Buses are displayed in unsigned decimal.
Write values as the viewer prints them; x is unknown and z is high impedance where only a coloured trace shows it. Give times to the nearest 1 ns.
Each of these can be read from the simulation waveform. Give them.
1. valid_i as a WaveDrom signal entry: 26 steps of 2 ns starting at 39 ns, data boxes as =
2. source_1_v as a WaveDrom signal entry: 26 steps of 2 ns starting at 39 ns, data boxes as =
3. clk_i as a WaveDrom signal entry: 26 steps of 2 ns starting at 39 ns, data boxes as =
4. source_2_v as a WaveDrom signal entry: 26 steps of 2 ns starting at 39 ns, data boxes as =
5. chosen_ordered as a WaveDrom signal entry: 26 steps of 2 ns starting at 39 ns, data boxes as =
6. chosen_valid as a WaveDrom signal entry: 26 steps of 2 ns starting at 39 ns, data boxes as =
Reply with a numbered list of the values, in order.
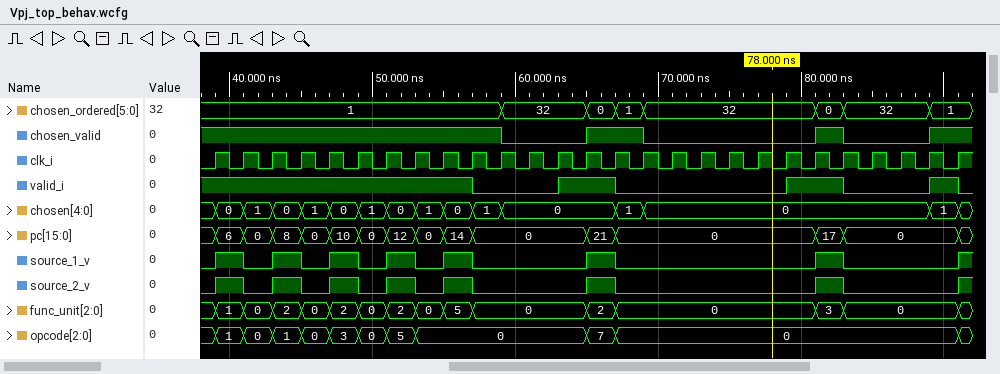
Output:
1. {name: 'valid_i', wave: '1........0..1.0.....1.0..1'}
2. {name: 'source_1_v', wave: '1010101010...10......10...'}
3. {name: 'clk_i', wave: 'p.........................'}
4. {name: 'source_2_v', wave: '1010101010...10......10...'}
5. {name: 'chosen_ordered', wave: '=.........=..===.....==..=', data: '1 32 0 1 32 0 32 1'}
6. {name: 'chosen_valid', wave: '1.........0..1.0.....10..1'}
